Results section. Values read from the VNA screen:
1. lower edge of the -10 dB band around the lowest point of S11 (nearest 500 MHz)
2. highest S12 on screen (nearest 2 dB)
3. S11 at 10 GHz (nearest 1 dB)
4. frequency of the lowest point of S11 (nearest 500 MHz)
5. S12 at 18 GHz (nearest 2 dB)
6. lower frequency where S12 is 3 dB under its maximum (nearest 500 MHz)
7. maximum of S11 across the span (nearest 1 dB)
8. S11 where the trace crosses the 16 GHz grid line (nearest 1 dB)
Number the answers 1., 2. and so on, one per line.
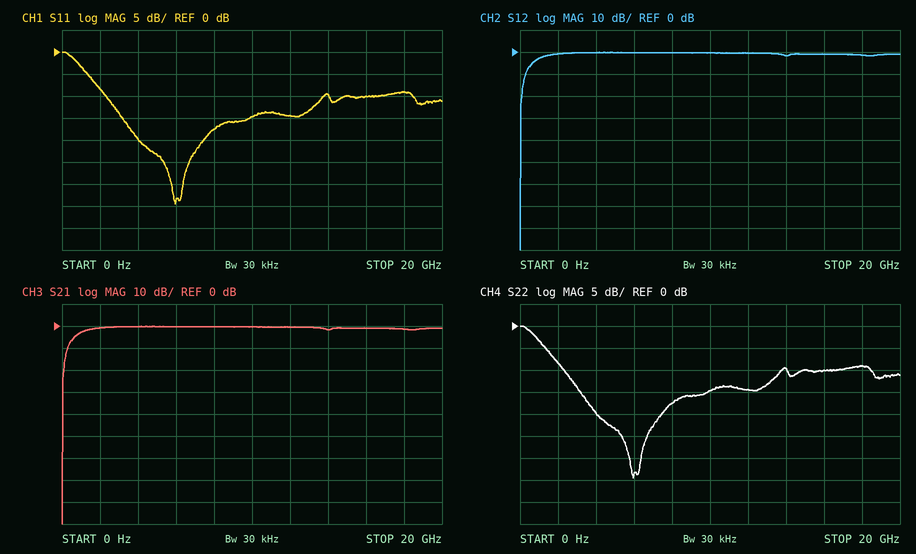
1. 2.5 GHz
2. 0 dB
3. -15 dB
4. 6.0 GHz
5. -2 dB
6. 1.0 GHz
7. 0 dB
8. -10 dB
